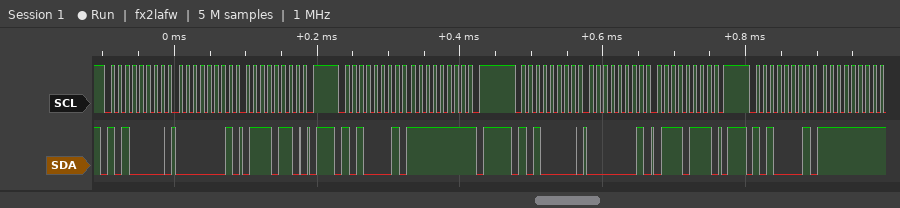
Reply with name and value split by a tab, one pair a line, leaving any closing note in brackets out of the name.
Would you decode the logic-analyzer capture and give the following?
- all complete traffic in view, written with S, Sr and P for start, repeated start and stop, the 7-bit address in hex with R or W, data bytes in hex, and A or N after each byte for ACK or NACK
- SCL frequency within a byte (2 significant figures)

all complete traffic in view, written with S, Sr and P for start, repeated start and stop, the 7-bit address in hex with R or W, data bytes in hex, and A or N after each byte for ACK or NACK	S 50W A 01 A 76 A P S 50R A FF N P S 50W A 01 A 77 A P S 50R A FF N
SCL frequency within a byte	100 kHz
